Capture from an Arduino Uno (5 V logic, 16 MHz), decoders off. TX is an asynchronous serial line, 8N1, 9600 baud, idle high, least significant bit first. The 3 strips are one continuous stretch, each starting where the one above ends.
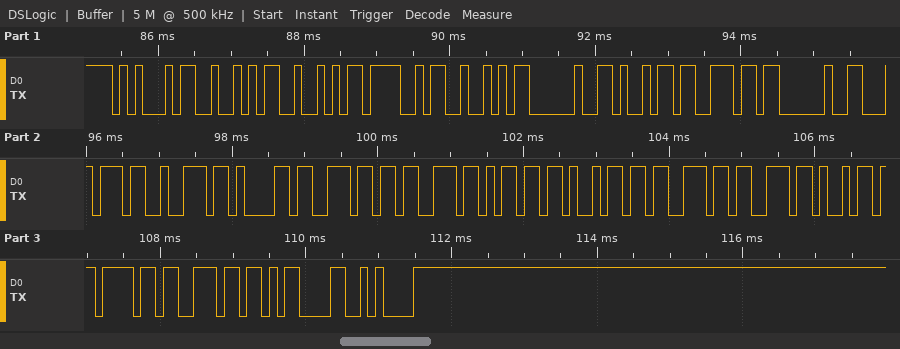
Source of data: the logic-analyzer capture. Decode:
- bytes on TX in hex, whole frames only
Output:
0x45 0x52 0x52 0x4F 0x52 0x20 0x69 0x6E 0x20 0x74 0x72 0x61 0x6E 0x73 0x6D 0x69 0x73 0x73 0x69 0x6F 0x6E 0x0D 0x0A
